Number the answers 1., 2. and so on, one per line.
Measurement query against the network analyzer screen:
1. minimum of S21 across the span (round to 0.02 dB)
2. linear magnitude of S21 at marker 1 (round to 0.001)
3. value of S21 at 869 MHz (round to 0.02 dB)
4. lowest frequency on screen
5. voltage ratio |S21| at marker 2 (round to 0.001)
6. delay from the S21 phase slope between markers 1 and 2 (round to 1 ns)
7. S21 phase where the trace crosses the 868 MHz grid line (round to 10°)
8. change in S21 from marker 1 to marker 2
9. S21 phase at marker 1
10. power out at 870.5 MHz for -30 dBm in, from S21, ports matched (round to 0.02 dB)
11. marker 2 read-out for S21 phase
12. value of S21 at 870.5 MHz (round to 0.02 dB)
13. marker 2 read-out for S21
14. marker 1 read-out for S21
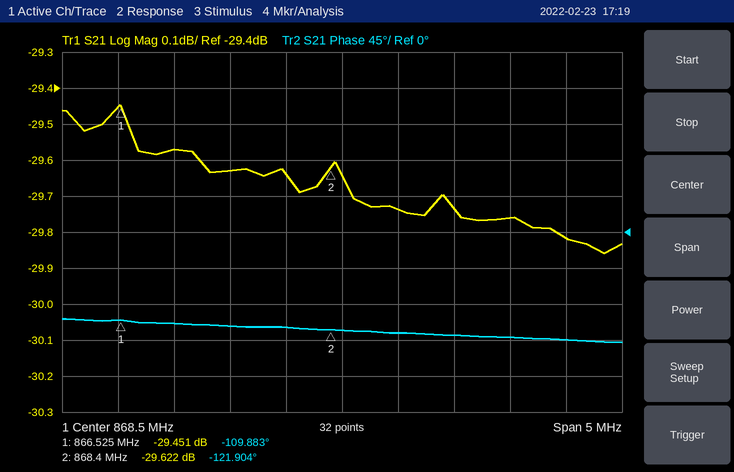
1. -29.86 dB
2. 0.034
3. -29.74 dB
4. 866 MHz
5. 0.033
6. 18 ns
7. -120°
8. -0.171 dB
9. -109.883°
10. -59.82 dBm
11. -121.904°
12. -29.82 dB
13. -29.622 dB
14. -29.451 dB
